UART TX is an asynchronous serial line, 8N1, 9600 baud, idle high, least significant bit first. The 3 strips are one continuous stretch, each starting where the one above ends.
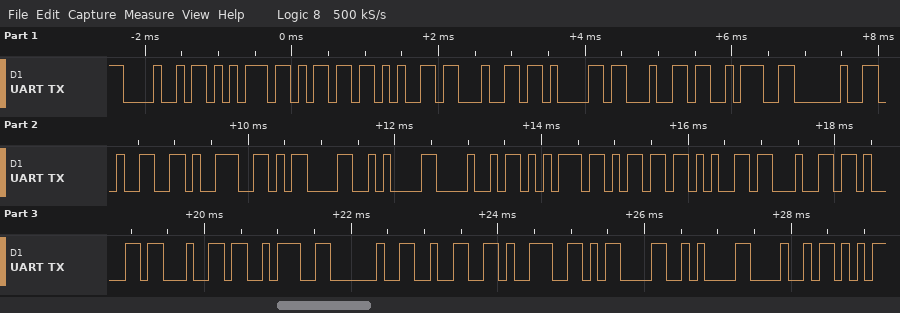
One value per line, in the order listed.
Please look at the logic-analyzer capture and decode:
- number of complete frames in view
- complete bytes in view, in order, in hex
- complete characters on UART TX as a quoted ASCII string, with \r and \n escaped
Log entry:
27
48 75 6D 65 64 61 64 3A 20 32 39 0D 0A 48 75 6D 65 64 61 64 3A 20 32 39 0D 0A 48
"Humedad: 29\r\nHumedad: 29\r\nH"
